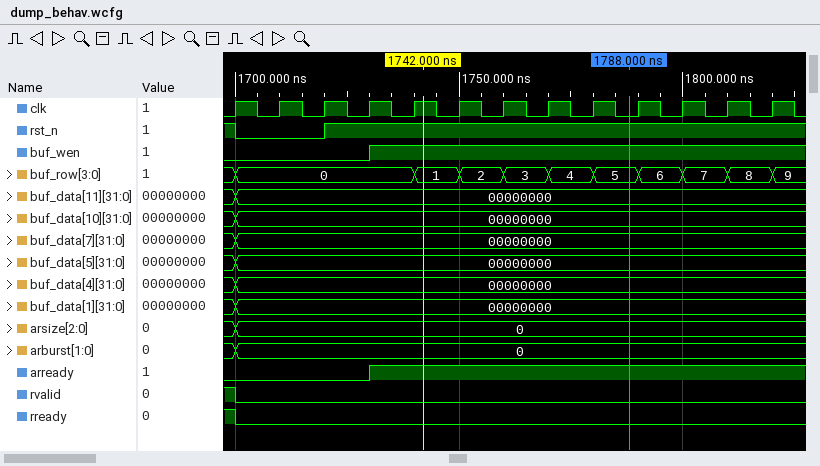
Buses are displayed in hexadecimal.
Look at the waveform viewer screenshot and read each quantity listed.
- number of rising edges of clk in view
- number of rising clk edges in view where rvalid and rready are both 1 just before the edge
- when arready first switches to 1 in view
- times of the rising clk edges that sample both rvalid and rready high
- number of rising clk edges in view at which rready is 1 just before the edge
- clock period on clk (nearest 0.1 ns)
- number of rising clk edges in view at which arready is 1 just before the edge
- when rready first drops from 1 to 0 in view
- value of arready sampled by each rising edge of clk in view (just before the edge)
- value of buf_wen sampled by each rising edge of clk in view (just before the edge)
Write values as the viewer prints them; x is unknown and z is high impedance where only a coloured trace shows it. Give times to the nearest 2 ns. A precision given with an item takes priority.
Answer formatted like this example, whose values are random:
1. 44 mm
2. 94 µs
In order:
1. 13
2. 1
3. 1730 ns
4. 1700 ns
5. 1
6. 10 ns
7. 9
8. 1700 ns
9. 0 0 0 0 1 1 1 1 1 1 1 1 1
10. 0 0 0 0 1 1 1 1 1 1 1 1 1
